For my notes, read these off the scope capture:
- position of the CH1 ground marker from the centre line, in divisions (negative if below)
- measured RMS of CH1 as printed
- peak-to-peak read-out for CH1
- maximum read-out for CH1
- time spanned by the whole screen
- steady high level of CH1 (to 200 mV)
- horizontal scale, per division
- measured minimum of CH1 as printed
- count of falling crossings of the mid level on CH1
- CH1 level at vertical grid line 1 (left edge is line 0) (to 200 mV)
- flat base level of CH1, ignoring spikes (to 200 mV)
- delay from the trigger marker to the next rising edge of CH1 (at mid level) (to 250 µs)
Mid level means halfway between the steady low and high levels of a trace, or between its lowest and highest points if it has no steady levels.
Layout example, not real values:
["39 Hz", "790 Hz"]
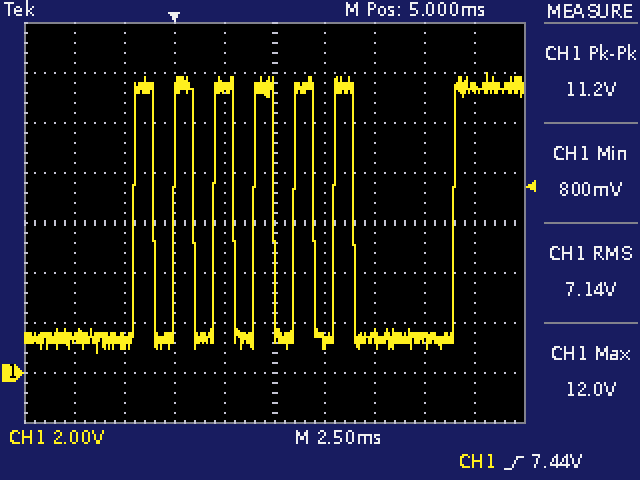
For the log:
["-3.0 div", "7.14 V", "11.2 V", "12.0 V", "25 ms", "11.4 V", "2.5 ms", "800 mV", "6", "1.4 V", "1.4 V", "2.00 ms"]
